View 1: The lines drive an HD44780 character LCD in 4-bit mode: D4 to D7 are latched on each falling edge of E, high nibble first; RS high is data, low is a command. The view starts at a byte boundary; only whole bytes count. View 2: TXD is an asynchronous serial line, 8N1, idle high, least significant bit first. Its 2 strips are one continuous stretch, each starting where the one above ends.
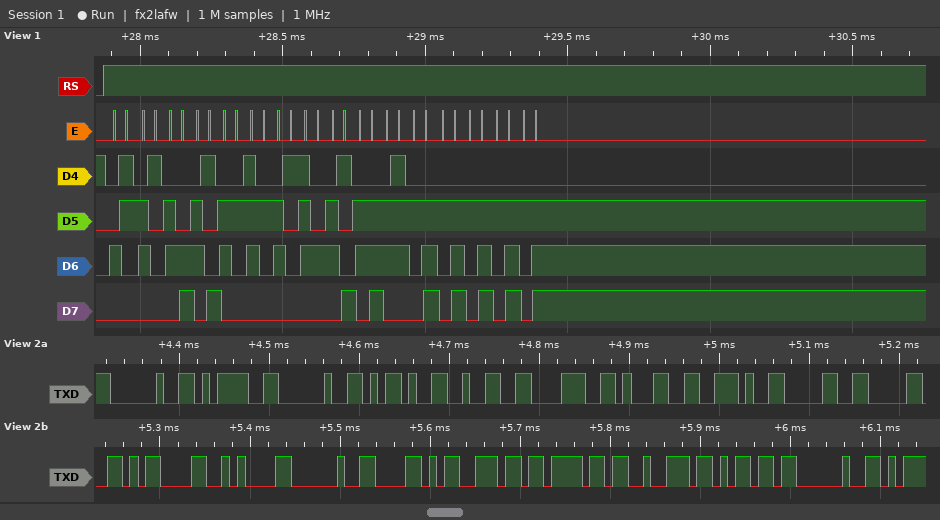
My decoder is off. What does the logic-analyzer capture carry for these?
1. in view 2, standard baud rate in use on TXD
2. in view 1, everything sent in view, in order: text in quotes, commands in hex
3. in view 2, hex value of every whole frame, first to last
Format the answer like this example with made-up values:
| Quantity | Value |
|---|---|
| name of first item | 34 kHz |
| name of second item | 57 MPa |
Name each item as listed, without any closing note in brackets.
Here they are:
| Quantity | Value |
|---|---|
| in view 2, standard baud rate in use on TXD | 115200 baud |
| in view 1, everything sent in view, in order: text in quotes, commands in hex | "Calibrating....." |
| in view 2, hex value of every whole frame, first to last | 20 3D 20 2D 32 38 31 2E 30 30 0D 0A 20 58 6E 6F 72 6D 20 |
